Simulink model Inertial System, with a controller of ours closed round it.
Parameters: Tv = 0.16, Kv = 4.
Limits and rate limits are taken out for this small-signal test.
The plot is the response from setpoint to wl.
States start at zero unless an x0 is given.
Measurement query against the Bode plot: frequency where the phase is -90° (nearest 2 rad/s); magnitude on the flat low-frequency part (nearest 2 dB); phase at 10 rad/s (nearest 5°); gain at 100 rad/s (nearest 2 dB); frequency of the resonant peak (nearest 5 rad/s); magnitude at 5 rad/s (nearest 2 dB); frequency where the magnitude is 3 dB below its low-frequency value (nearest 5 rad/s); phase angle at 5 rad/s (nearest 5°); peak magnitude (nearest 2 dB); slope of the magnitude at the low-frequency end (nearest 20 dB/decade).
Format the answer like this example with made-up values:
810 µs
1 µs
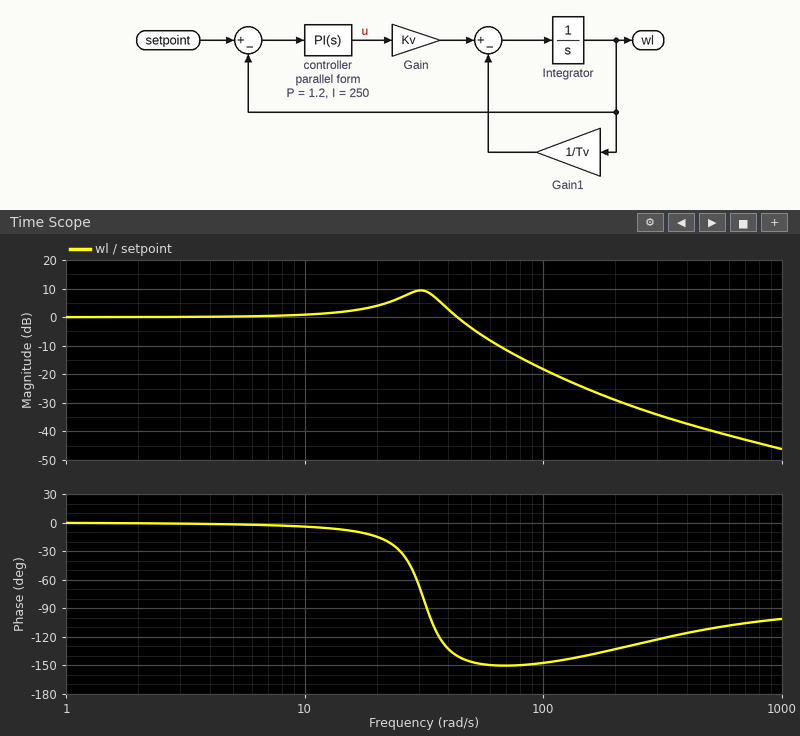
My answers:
32 rad/s
0 dB
-5°
-18 dB
30 rad/s
0 dB
50 rad/s
0°
10 dB
0 dB/decade
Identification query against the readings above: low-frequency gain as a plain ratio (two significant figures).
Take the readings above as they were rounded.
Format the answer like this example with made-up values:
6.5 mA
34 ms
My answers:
1.0
